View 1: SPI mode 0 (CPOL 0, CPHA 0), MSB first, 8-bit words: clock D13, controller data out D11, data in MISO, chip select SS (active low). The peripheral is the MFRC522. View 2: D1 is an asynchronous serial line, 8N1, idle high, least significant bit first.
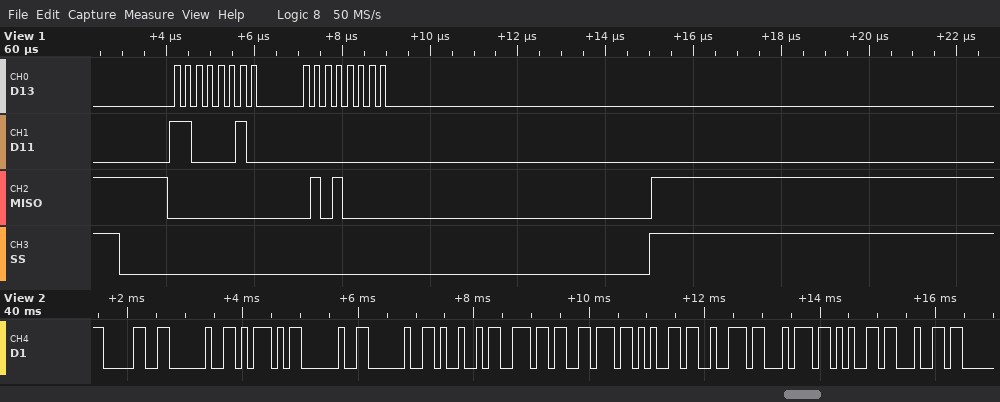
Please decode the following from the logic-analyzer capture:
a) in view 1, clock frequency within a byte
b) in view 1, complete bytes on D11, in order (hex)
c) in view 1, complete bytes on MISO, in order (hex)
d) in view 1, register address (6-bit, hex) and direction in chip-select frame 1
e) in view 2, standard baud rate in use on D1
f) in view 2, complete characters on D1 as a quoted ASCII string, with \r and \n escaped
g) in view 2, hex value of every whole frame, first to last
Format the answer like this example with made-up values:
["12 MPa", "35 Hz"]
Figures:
["4 MHz", "C2 00", "00 50", "0x21 read", "9600 baud", "\"0 ]  Inverted\"", "30 20 5D 20 20 49 6E 76 65 72 74 65 64"]
